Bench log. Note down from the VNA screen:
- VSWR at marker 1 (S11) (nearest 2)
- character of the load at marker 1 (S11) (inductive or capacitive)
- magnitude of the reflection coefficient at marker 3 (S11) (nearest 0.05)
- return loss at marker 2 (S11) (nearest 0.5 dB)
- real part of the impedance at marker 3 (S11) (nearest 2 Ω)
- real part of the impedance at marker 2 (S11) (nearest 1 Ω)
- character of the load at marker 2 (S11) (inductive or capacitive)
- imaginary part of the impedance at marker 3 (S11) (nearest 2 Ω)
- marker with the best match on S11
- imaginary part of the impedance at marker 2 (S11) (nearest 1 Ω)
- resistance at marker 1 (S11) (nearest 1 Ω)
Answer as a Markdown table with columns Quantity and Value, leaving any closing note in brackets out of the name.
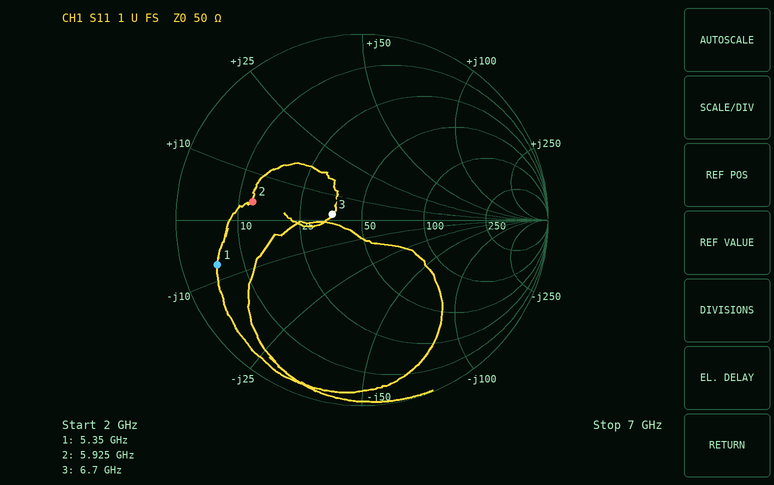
| Quantity | Value |
|---|---|
| VSWR at marker 1 (S11) | 10 |
| character of the load at marker 1 (S11) | capacitive |
| magnitude of the reflection coefficient at marker 3 (S11) | 0.15 |
| return loss at marker 2 (S11) | 4.5 dB |
| real part of the impedance at marker 3 (S11) | 36 Ω |
| real part of the impedance at marker 2 (S11) | 13 Ω |
| character of the load at marker 2 (S11) | inductive |
| imaginary part of the impedance at marker 3 (S11) | +2 Ω |
| marker with the best match on S11 | marker 3 |
| imaginary part of the impedance at marker 2 (S11) | +4 Ω |
| resistance at marker 1 (S11) | 5 Ω |
